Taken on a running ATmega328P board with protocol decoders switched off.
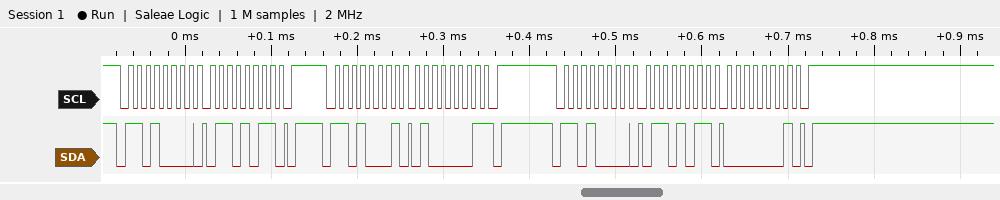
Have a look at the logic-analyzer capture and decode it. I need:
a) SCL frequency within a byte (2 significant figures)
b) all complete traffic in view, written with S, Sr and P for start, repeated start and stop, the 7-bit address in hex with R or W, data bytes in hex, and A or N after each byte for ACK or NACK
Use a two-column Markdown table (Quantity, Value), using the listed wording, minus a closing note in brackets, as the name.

| Quantity | Value |
|---|---|
| SCL frequency within a byte | 100 kHz |
| all complete traffic in view, written with S, Sr and P for start, repeated start and stop, the 7-bit address in hex with R or W, data bytes in hex, and A or N after each byte for ACK or NACK | S 68W A 6B A P S 68R A 41 N P S 68W A 6B A 01 A P |
